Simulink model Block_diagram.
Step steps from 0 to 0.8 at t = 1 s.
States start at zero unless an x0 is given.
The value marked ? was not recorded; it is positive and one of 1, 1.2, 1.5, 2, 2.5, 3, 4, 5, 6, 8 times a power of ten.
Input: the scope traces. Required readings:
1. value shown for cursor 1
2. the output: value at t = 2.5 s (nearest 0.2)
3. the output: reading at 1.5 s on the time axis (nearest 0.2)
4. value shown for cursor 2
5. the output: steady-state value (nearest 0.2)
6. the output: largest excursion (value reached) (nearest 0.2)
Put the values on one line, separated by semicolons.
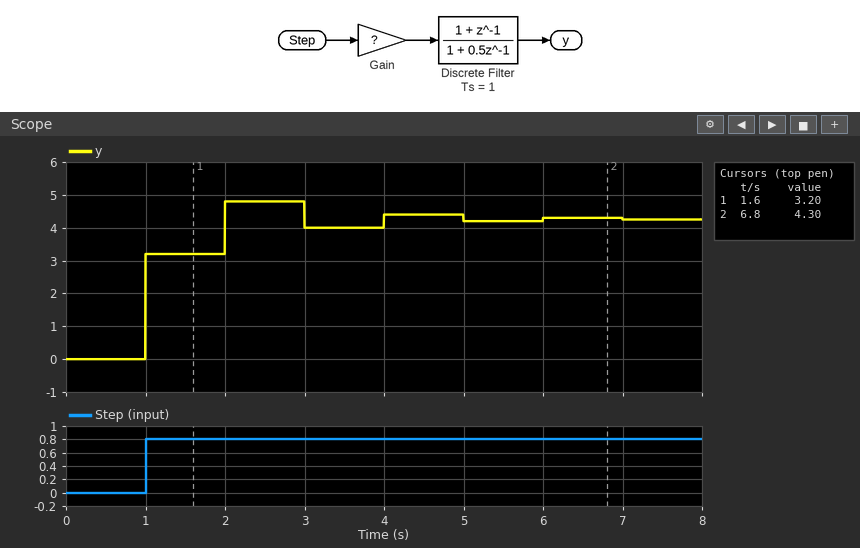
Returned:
3.20; 4.8; 3.2; 4.30; 4.2; 4.8
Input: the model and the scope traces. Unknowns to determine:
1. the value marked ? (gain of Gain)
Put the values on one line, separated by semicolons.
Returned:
4
